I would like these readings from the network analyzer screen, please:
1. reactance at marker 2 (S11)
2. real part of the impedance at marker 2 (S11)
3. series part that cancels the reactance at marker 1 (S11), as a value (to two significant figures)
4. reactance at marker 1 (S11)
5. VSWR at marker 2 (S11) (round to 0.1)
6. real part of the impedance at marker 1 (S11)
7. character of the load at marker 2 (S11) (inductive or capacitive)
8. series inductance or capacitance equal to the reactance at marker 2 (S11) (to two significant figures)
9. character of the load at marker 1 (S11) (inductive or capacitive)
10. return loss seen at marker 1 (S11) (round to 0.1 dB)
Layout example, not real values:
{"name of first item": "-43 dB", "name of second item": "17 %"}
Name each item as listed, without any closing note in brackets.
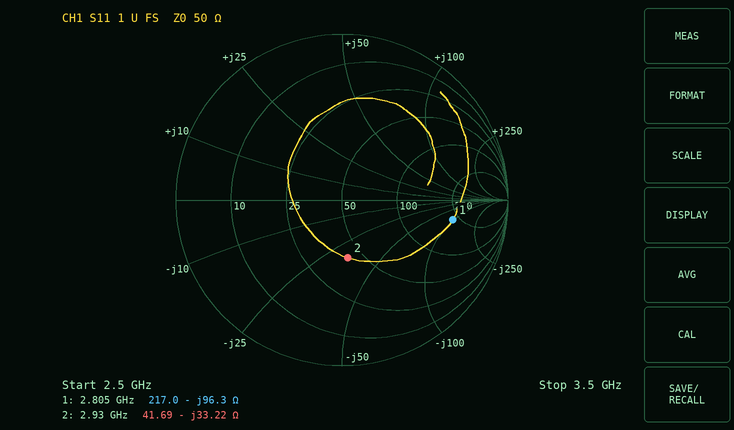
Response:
{"reactance at marker 2": "-33.22 Ω", "real part of the impedance at marker 2": "41.69 Ω", "series part that cancels the reactance at marker 1 (S11), as a value": "5.5 nH", "reactance at marker 1": "-96.3 Ω", "VSWR at marker 2 (S11)": "2.1", "real part of the impedance at marker 1": "217.0 Ω", "character of the load at marker 2 (S11)": "capacitive", "series inductance or capacitance equal to the reactance at marker 2 (S11)": "1.6 pF", "character of the load at marker 1 (S11)": "capacitive", "return loss seen at marker 1 (S11)": "3.4 dB"}
